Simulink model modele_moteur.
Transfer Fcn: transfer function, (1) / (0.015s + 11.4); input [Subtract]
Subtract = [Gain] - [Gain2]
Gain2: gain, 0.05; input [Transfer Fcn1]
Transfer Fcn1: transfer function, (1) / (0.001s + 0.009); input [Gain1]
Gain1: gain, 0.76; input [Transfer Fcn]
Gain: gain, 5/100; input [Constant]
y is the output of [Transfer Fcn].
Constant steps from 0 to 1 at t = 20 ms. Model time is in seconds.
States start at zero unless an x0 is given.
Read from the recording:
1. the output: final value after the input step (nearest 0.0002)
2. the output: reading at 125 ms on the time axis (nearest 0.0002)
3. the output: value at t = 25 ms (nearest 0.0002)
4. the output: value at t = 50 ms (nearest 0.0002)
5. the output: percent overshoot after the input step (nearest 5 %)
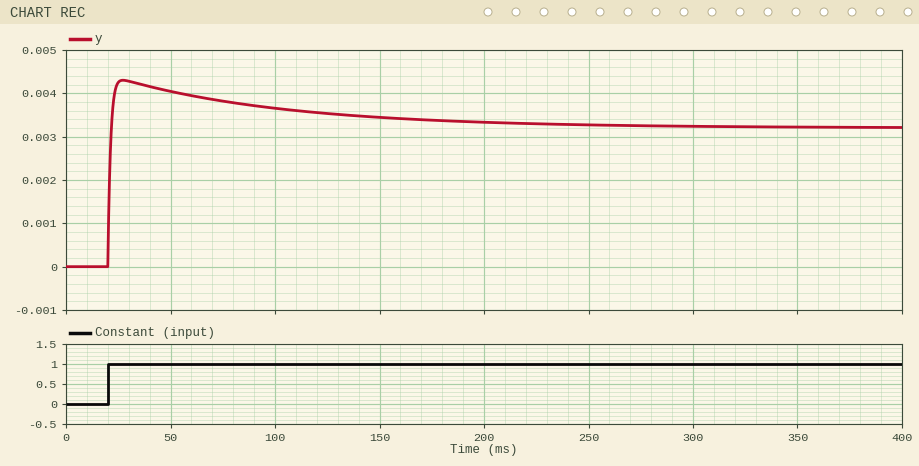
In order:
0.0032
0.0036
0.0042
0.0040
35 %
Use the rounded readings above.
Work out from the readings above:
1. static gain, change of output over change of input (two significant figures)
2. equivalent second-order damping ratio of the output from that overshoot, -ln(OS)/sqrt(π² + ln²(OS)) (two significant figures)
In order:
0.0032
0.32
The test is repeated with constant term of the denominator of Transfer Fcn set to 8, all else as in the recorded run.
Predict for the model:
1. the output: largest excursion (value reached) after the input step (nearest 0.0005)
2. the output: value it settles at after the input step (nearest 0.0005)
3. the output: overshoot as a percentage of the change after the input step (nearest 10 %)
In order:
0.0060
0.0040
50 %
